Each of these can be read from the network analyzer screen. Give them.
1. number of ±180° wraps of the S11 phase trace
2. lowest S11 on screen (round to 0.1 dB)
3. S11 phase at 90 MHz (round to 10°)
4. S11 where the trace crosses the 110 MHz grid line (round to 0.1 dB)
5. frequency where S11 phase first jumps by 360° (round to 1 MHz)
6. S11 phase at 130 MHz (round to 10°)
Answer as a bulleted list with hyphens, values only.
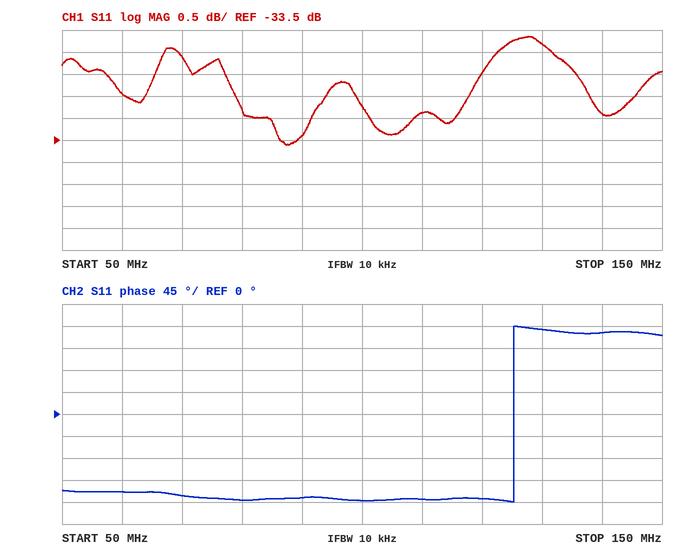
- 1
- -33.6 dB
- -170°
- -32.9 dB
- 125 MHz
- 170°
